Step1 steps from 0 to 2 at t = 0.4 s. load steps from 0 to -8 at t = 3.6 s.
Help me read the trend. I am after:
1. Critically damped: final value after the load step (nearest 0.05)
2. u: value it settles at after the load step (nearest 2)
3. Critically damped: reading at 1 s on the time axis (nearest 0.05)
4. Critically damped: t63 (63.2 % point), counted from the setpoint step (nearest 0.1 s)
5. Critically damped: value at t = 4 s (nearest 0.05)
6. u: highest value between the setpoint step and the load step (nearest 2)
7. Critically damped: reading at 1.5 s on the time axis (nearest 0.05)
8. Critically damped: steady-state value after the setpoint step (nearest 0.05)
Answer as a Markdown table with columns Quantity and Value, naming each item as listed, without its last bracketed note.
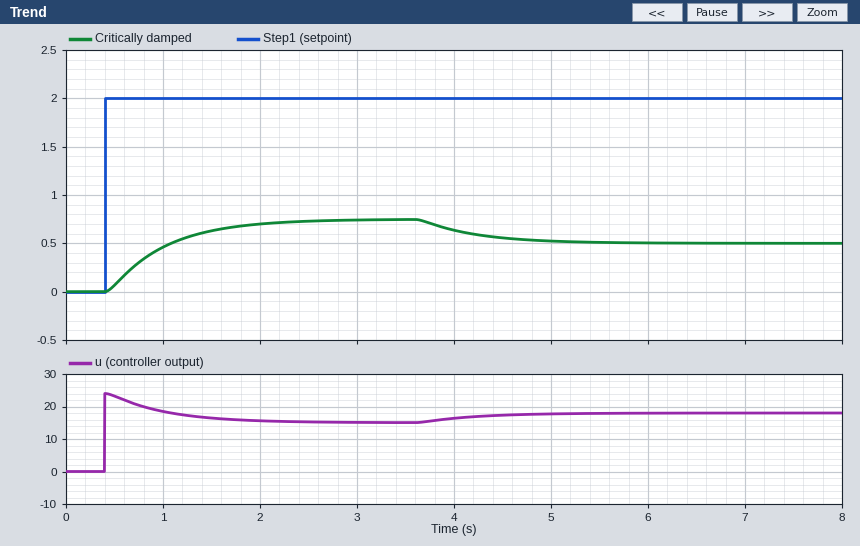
| Quantity | Value |
|---|---|
| Critically damped: final value after the load step | 0.50 |
| u: value it settles at after the load step | 18 |
| Critically damped: reading at 1 s on the time axis | 0.45 |
| Critically damped: t63 (63.2 % point), counted from the setpoint step | 0.6 s |
| Critically damped: value at t = 4 s | 0.65 |
| u: highest value between the setpoint step and the load step | 24 |
| Critically damped: reading at 1.5 s on the time axis | 0.65 |
| Critically damped: steady-state value after the setpoint step | 0.75 |
